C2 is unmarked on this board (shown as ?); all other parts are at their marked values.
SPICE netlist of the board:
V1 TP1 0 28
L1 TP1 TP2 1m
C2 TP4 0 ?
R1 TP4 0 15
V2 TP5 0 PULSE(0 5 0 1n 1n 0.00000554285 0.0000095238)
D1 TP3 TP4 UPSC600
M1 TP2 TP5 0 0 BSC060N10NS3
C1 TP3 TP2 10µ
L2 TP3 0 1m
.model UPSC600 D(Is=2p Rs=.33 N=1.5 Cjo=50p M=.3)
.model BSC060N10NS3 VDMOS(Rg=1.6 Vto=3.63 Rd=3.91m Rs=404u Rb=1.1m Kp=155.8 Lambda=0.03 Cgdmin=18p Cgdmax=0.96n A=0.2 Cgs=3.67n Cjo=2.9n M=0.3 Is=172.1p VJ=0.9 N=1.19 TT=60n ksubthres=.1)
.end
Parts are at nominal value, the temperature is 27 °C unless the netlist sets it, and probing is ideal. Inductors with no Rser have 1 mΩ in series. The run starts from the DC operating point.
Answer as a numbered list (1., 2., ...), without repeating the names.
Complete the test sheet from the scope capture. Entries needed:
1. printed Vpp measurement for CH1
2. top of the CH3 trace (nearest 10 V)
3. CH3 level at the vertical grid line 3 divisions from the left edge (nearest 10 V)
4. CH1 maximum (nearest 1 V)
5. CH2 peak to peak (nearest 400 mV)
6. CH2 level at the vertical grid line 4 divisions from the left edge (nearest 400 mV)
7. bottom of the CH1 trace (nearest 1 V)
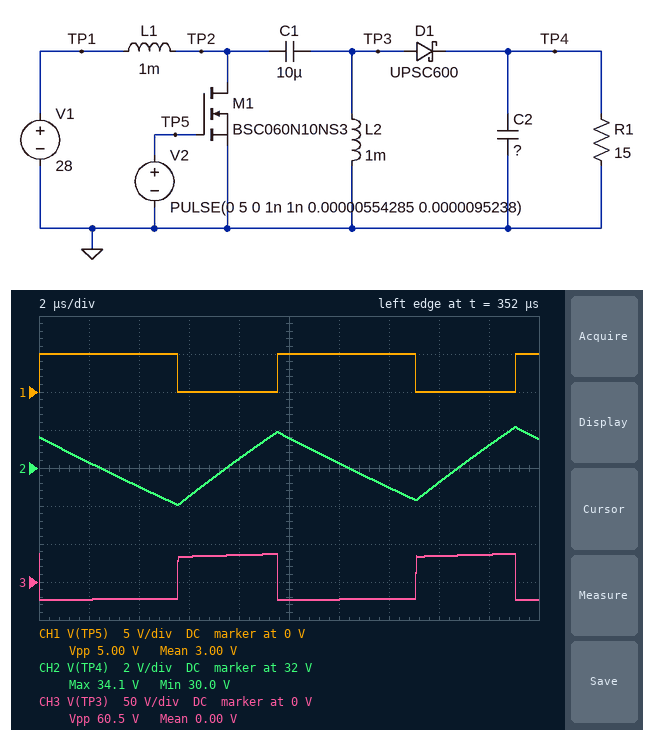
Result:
1. 5.00 V
2. 40 V
3. 30 V
4. 5 V
5. 4.0 V
6. 32.4 V
7. 0 V
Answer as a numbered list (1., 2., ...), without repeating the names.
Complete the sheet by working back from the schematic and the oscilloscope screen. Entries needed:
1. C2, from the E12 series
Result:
1. 3.3 µF
